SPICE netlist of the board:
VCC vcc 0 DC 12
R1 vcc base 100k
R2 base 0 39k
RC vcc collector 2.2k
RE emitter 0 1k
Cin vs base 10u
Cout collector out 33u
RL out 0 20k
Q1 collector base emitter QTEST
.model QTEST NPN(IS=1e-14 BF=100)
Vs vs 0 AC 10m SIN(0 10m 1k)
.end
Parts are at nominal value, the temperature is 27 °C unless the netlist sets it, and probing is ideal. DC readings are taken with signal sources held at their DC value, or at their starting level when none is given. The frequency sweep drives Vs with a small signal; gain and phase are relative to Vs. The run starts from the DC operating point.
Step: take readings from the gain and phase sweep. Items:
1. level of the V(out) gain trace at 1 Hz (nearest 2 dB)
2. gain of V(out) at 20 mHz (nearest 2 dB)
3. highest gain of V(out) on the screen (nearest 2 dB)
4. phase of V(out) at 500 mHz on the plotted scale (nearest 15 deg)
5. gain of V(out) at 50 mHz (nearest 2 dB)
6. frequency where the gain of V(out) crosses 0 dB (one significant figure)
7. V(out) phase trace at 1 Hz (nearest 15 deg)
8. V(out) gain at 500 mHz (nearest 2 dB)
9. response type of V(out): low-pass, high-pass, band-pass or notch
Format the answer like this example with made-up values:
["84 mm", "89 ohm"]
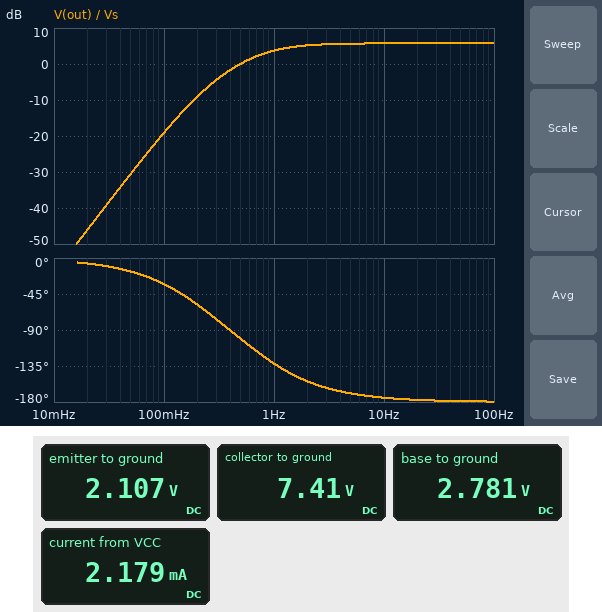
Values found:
["4 dB", "-46 dB", "6 dB", "-105 deg", "-30 dB", "500 mHz", "-135 deg", "0 dB", "high-pass"]
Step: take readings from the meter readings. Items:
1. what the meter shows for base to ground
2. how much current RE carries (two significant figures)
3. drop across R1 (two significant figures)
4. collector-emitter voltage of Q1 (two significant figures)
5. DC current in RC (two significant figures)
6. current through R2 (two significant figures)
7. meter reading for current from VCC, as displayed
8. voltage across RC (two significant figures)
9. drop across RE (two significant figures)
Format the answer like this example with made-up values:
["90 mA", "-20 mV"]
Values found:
["2.781 V", "2.1 mA", "9.2 V", "5.3 V", "2.1 mA", "71 µA", "2.179 mA", "4.6 V", "2.1 V"]
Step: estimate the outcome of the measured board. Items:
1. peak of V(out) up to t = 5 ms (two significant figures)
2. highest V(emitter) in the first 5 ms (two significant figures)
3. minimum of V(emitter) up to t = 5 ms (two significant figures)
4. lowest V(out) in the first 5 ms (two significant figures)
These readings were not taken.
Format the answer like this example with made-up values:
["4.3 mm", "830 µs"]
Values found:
["19 mV", "2.1 V", "2.1 V", "-19 mV"]
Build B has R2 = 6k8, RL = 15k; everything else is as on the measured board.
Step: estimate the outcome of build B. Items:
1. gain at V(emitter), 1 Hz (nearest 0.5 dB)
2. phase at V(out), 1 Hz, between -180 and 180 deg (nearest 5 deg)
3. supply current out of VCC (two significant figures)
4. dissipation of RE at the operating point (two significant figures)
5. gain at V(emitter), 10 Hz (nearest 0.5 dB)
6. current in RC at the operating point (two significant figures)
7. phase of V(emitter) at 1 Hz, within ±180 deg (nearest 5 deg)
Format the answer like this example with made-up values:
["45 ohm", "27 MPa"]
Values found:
["-10.5 dB", "-95 deg", "260 µA", "22 µW", "-1.5 dB", "150 µA", "70 deg"]
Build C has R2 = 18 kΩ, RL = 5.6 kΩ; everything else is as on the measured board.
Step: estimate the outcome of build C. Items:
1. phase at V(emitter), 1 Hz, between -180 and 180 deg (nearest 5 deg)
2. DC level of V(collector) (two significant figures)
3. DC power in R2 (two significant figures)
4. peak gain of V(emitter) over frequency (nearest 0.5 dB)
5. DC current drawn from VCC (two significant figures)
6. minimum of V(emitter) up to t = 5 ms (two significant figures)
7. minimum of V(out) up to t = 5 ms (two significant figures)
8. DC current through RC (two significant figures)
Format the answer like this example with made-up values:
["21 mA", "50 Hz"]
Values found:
["50 deg", "9.8 V", "160 µW", "0 dB", "1.1 mA", "1.0 V", "-15 mV", "1.0 mA"]
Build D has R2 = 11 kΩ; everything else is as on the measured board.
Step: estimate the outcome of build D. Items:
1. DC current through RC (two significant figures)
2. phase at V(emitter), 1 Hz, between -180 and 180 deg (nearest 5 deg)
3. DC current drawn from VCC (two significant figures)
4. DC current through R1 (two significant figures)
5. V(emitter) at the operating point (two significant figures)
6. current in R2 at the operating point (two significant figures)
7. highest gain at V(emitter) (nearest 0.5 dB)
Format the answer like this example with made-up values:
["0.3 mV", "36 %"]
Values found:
["500 µA", "60 deg", "610 µA", "110 µA", "500 mV", "100 µA", "-0.5 dB"]
